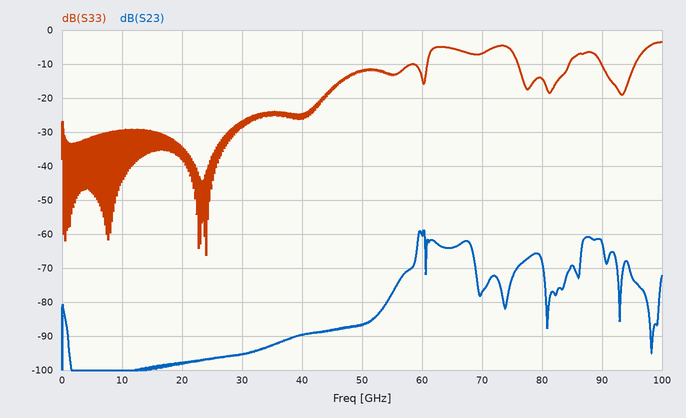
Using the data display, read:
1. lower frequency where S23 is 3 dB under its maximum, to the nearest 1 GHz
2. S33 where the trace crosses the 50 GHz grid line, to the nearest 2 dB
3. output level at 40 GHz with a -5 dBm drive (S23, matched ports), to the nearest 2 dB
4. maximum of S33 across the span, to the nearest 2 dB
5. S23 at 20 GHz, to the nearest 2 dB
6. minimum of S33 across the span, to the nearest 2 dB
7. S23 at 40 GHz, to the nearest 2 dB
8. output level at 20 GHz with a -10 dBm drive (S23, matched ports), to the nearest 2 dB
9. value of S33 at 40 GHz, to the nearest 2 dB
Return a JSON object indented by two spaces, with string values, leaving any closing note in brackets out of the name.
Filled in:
{
  "lower frequency where S23 is 3 dB under its maximum, to the nearest 1 GHz": "59 GHz",
  "S33 where the trace crosses the 50 GHz grid line, to the nearest 2 dB": "-12 dB",
  "output level at 40 GHz with a -5 dBm drive (S23, matched ports), to the nearest 2 dB": "-94 dBm",
  "maximum of S33 across the span, to the nearest 2 dB": "-4 dB",
  "S23 at 20 GHz, to the nearest 2 dB": "-98 dB",
  "minimum of S33 across the span, to the nearest 2 dB": "-66 dB",
  "S23 at 40 GHz, to the nearest 2 dB": "-90 dB",
  "output level at 20 GHz with a -10 dBm drive (S23, matched ports), to the nearest 2 dB": "-108 dBm",
  "value of S33 at 40 GHz, to the nearest 2 dB": "-26 dB"
}
